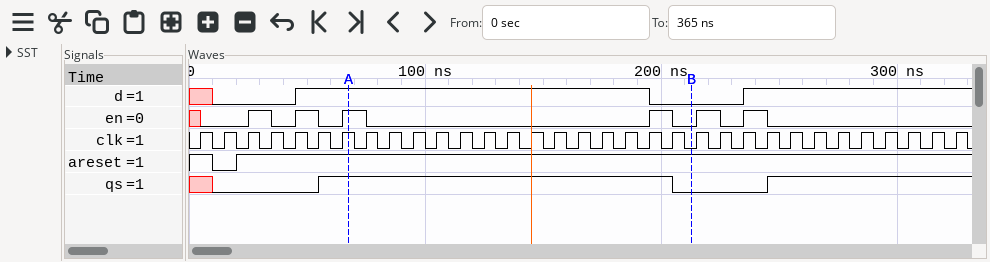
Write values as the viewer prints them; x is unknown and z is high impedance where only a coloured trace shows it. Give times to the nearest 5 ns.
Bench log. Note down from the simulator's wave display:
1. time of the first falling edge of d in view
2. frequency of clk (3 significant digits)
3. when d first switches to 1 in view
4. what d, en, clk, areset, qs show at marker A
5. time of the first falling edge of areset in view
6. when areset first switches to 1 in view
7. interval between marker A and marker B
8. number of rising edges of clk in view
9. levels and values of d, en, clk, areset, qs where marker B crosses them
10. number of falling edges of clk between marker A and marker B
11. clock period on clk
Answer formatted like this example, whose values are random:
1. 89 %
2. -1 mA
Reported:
1. 195 ns
2. 100 MHz
3. 45 ns
4. d=1, en=1, clk=1, areset=1, qs=1
5. 10 ns
6. 20 ns
7. 145 ns
8. 33
9. d=0, en=0, clk=0, areset=1, qs=0
10. 15
11. 10 ns
